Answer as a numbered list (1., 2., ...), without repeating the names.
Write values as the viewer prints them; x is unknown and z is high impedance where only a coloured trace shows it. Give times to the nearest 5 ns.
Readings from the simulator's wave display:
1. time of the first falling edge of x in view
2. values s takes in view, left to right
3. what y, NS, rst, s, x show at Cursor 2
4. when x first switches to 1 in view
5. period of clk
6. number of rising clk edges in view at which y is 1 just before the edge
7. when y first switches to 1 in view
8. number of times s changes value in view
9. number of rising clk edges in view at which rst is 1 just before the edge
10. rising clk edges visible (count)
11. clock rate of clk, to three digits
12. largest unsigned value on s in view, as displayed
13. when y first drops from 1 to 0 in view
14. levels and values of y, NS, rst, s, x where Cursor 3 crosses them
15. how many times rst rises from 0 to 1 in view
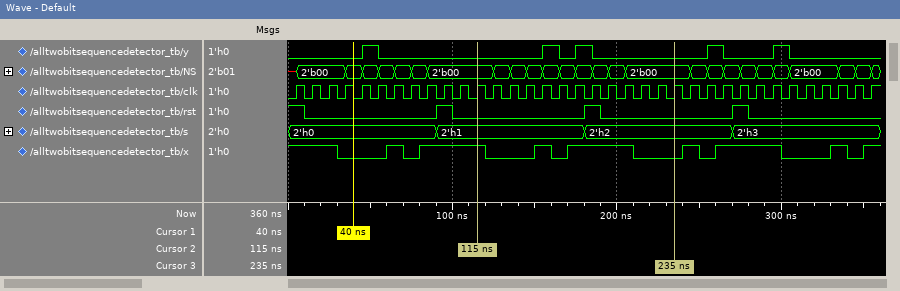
1. 30 ns
2. 2'h0, 2'h1, 2'h2, 2'h3
3. y=0, NS=2'b00, rst=0, s=2'h1, x=1
4. 60 ns
5. 10 ns
6. 5
7. 45 ns
8. 3
9. 4
10. 36
11. 100 MHz
12. 2'h3
13. 55 ns
14. y=0, NS=2'b00, rst=0, s=2'h2, x=0
15. 3
